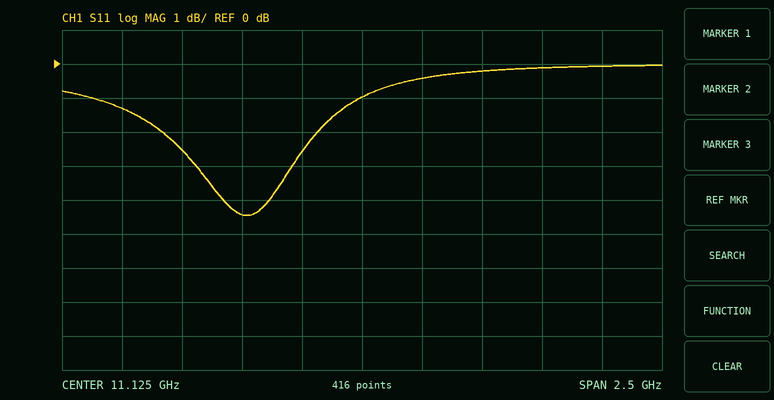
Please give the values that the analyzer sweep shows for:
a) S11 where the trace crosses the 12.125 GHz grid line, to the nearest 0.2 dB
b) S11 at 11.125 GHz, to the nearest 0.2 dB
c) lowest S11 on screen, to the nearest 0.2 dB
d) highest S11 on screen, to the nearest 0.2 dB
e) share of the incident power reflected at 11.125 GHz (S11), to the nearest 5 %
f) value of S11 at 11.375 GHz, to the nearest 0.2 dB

0.0 dB
-1.0 dB
-4.4 dB
0.0 dB
80 %
-0.4 dB
